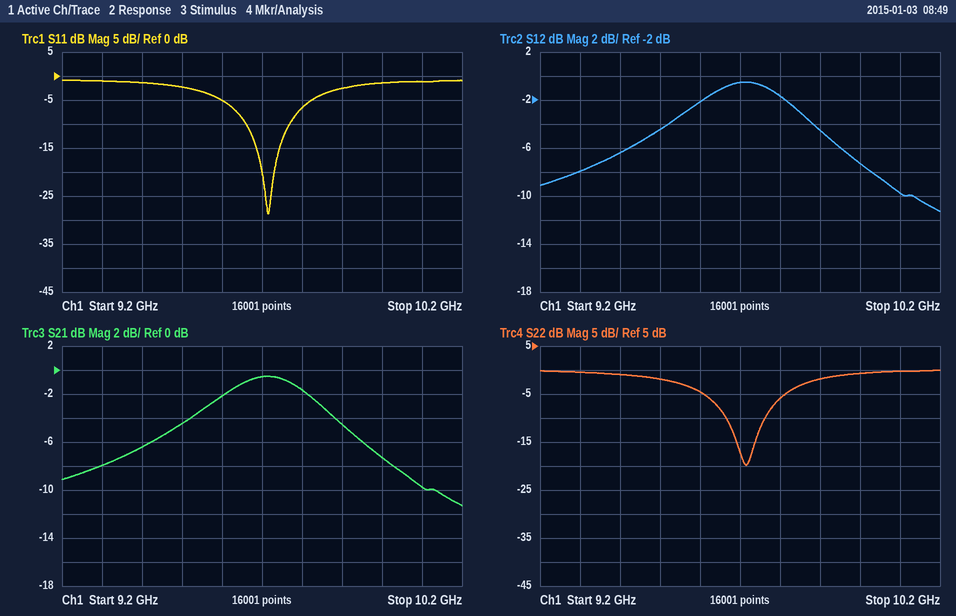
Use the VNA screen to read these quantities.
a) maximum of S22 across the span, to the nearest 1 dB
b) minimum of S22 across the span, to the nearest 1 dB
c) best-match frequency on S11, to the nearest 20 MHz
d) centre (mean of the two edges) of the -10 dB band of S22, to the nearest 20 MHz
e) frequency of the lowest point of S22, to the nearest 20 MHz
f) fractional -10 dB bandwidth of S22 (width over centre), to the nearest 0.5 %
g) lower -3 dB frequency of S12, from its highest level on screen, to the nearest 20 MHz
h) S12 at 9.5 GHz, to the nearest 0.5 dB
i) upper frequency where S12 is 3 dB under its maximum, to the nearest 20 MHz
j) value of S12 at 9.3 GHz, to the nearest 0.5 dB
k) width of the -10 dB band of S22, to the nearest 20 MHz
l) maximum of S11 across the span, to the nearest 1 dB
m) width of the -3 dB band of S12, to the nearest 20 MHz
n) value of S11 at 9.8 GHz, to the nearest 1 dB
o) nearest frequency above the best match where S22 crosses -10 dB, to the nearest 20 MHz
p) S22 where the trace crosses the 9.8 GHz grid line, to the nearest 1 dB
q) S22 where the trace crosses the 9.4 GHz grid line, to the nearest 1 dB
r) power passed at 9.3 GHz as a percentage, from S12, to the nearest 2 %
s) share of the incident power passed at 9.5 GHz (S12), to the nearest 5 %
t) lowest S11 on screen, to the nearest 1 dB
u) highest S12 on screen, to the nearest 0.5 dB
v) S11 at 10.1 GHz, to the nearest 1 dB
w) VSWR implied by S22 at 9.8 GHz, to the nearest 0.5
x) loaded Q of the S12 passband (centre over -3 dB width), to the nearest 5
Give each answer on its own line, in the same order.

0 dB
-20 dB
9.72 GHz
9.72 GHz
9.72 GHz
1.0 %
9.54 GHz
-4.5 dB
9.86 GHz
-8.0 dB
100 MHz
-1 dB
320 MHz
-7 dB
9.76 GHz
-6 dB
-1 dB
16 %
35 %
-29 dB
-0.5 dB
-1 dB
3.0
30
